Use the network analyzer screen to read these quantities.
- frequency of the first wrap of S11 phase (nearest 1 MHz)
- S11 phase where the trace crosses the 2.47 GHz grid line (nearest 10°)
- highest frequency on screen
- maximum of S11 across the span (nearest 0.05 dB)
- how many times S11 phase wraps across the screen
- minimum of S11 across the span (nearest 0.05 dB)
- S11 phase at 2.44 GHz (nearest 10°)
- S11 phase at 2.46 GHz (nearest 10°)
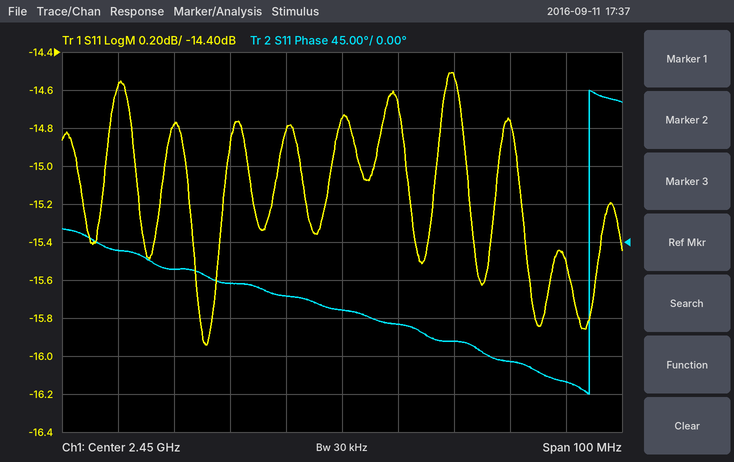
2.494 GHz
-120°
2.5 GHz
-14.50 dB
1
-15.95 dB
-60°
-100°
